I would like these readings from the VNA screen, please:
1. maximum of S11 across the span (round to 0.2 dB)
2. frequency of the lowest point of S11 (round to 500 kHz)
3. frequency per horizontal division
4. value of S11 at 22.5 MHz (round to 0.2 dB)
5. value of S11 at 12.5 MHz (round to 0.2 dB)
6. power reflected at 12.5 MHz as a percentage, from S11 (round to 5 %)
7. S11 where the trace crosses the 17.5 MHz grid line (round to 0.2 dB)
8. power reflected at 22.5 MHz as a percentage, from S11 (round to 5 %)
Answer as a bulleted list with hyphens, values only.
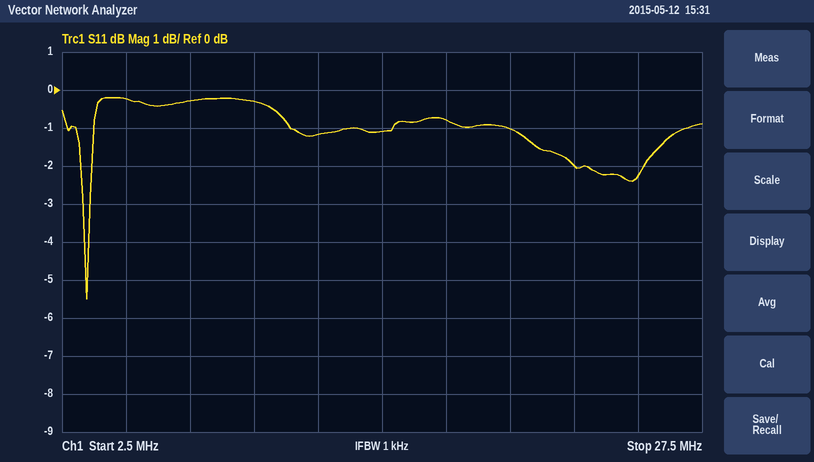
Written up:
- -0.2 dB
- 3.5 MHz
- 2.5 MHz
- -2.0 dB
- -1.2 dB
- 75 %
- -0.8 dB
- 65 %
